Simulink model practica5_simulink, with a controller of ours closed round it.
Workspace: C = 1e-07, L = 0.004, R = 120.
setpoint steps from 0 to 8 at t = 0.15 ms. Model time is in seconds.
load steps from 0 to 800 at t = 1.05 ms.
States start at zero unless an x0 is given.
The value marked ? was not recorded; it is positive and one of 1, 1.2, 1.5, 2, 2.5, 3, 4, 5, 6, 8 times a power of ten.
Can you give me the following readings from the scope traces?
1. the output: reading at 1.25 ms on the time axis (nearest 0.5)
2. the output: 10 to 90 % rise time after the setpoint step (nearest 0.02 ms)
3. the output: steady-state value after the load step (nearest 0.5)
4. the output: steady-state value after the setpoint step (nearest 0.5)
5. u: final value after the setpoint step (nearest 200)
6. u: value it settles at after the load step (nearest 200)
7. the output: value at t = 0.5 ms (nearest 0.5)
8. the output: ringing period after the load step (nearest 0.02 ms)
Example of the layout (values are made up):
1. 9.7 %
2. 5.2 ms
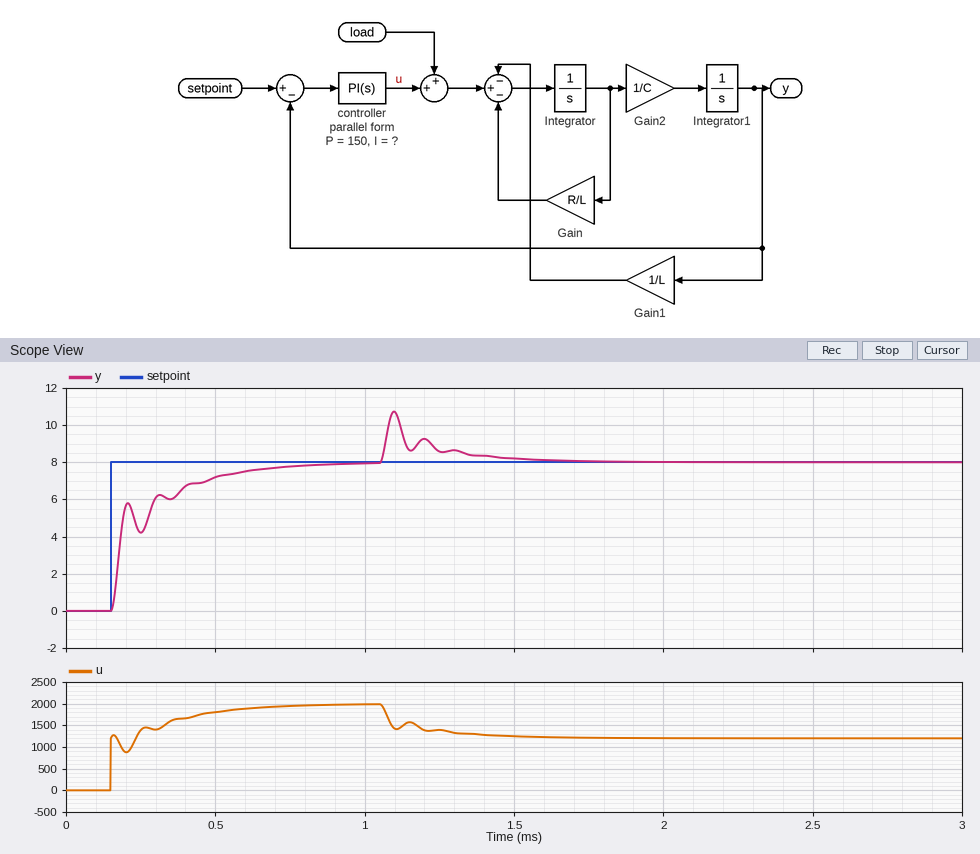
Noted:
1. 8.5
2. 0.34 ms
3. 8.0
4. 8.0
5. 2000
6. 1200
7. 7.0
8. 0.10 ms
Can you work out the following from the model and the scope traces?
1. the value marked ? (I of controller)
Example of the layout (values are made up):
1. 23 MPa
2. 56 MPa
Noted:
1. 2e+06
